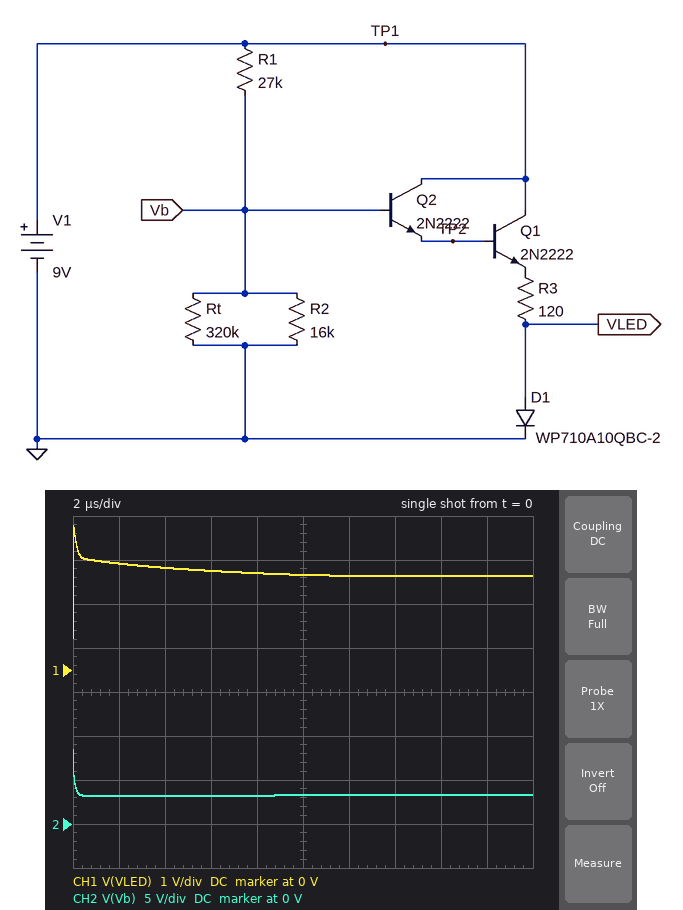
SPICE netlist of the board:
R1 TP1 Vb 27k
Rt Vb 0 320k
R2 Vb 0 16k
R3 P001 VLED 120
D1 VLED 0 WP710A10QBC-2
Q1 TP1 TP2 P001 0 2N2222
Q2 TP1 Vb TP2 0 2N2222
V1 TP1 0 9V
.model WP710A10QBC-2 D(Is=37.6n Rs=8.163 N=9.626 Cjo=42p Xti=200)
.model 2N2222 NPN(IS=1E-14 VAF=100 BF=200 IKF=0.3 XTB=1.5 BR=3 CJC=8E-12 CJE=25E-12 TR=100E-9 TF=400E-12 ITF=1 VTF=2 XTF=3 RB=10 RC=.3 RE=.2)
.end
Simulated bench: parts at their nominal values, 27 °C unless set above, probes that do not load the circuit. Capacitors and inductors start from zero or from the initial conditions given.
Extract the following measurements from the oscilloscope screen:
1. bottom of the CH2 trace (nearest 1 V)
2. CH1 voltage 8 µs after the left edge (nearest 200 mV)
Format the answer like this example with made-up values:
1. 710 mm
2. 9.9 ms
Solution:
1. 3 V
2. 2.2 V
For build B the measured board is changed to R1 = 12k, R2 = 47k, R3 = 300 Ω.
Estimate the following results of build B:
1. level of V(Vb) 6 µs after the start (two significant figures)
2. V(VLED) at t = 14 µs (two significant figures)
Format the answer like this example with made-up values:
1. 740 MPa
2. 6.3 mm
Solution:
1. 7.0 V
2. 3.1 V
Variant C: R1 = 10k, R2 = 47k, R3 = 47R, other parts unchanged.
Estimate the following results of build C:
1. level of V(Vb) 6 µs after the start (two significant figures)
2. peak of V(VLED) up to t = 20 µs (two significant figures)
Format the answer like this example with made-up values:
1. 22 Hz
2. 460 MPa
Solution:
1. 7.2 V
2. 3.8 V
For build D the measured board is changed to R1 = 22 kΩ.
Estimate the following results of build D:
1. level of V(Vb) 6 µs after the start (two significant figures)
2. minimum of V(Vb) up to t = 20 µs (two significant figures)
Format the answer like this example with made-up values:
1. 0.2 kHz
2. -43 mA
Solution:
1. 3.7 V
2. 3.6 V
